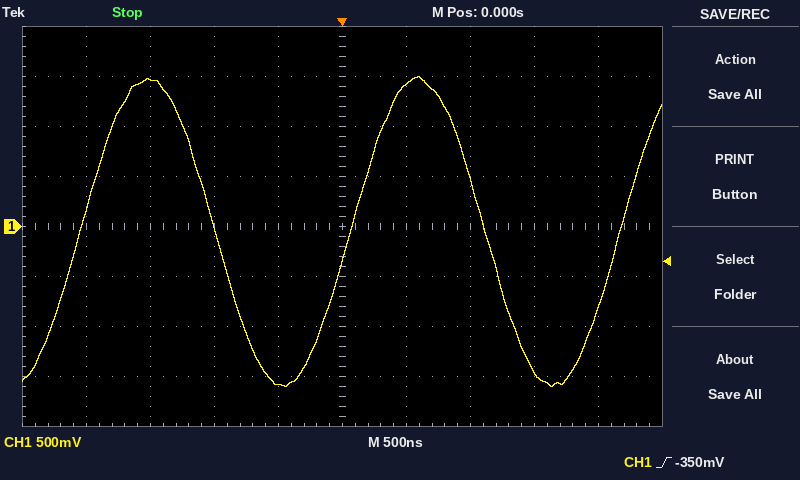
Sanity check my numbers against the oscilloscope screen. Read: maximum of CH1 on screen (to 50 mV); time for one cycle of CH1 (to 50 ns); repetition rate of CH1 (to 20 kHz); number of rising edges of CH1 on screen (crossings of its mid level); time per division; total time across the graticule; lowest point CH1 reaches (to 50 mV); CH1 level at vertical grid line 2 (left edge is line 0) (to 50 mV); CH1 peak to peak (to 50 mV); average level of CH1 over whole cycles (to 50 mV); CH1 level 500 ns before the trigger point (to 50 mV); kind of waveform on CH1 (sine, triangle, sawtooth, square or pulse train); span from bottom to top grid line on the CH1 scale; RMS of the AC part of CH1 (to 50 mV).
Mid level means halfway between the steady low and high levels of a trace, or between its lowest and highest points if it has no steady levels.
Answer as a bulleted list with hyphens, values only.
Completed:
- 1.50 V
- 2.10 µs
- 480 kHz
- 3
- 500 ns
- 5 µs
- -1.60 V
- 1.45 V
- 3.10 V
- -50 mV
- -1.60 V
- sine
- 4 V
- 1.10 V
